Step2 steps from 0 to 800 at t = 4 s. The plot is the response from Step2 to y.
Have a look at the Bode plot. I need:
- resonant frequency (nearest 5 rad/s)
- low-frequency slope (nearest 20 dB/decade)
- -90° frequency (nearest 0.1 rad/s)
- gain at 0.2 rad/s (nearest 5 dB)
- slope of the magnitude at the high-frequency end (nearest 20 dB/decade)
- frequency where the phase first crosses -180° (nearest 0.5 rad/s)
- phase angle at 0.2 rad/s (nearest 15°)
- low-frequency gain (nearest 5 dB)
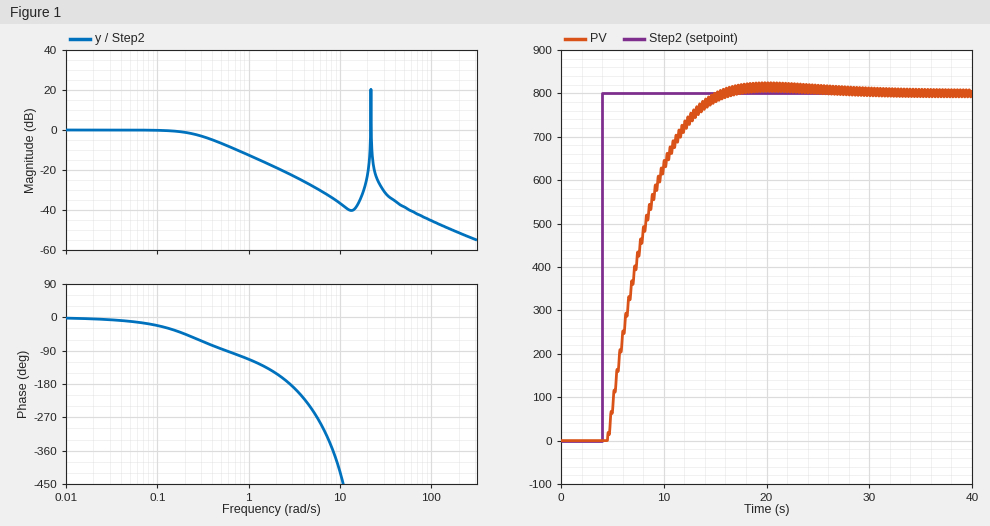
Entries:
20 rad/s
0 dB/decade
0.6 rad/s
0 dB
-20 dB/decade
3.0 rad/s
-45°
0 dB
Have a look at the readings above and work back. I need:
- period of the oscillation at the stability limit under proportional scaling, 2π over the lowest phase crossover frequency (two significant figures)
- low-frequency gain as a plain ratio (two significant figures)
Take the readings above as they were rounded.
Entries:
2.1 s
1.0
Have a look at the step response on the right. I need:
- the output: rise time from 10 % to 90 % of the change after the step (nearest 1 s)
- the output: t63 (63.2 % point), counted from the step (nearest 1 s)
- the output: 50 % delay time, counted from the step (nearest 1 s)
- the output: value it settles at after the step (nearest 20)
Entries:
7 s
4 s
3 s
800
